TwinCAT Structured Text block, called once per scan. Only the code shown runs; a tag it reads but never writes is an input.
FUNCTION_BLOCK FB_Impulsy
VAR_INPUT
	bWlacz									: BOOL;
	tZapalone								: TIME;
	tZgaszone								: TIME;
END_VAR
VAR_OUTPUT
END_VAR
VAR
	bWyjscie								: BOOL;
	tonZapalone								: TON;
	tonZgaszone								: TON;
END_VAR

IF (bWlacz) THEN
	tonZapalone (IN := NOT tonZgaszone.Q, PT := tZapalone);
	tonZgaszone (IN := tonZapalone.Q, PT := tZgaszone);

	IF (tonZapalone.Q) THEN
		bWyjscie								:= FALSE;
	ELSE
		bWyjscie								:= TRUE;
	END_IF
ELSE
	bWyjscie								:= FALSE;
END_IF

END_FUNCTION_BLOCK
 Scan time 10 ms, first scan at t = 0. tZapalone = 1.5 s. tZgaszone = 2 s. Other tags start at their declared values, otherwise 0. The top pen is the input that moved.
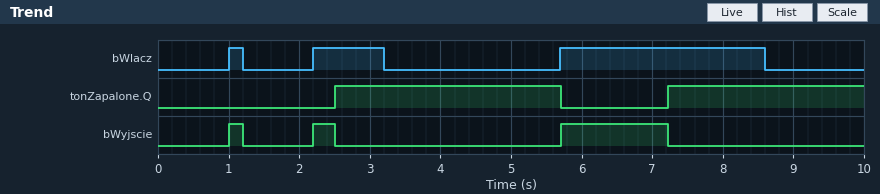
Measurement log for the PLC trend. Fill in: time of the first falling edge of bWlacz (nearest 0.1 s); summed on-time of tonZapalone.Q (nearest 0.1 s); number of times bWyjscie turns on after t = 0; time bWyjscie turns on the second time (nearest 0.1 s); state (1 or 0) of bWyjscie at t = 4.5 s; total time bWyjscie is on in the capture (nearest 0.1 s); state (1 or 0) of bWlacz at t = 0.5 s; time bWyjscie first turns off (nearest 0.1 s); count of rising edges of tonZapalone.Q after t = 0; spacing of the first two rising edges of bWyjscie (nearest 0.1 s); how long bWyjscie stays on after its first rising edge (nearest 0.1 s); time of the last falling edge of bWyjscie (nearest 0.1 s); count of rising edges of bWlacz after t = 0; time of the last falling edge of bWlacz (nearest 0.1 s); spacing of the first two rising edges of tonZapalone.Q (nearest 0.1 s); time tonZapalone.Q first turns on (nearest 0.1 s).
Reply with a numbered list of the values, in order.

1. 1.2 s
2. 6.0 s
3. 3
4. 2.2 s
5. 0
6. 2.0 s
7. 0
8. 1.2 s
9. 2
10. 1.2 s
11. 0.2 s
12. 7.2 s
13. 3
14. 8.6 s
15. 4.7 s
16. 2.5 s
